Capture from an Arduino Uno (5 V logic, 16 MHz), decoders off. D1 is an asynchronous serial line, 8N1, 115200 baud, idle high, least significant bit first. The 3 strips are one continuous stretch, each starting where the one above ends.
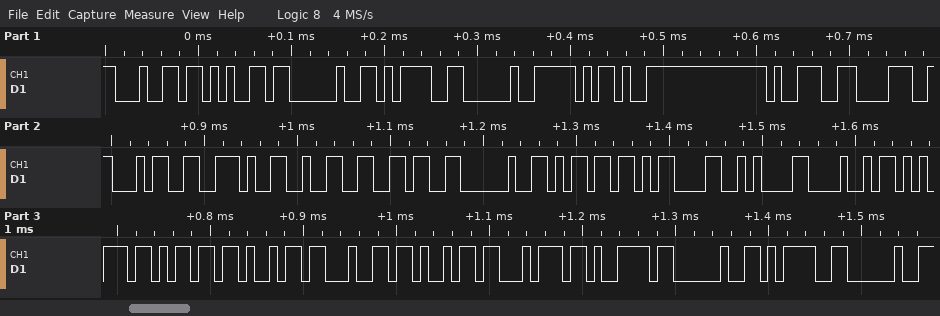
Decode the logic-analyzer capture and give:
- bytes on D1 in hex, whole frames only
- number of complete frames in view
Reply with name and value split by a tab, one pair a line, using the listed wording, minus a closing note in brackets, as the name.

bytes on D1 in hex, whole frames only	64 65 20 3D 20 2D 39 38 34 2E 32 36 20 6D 0D 0A 48 75 6D 69 64 69 74 79 20 3D 20
number of complete frames in view	27
